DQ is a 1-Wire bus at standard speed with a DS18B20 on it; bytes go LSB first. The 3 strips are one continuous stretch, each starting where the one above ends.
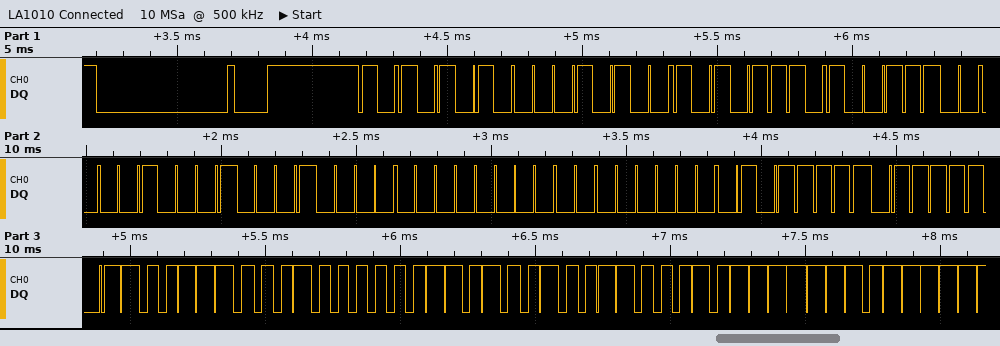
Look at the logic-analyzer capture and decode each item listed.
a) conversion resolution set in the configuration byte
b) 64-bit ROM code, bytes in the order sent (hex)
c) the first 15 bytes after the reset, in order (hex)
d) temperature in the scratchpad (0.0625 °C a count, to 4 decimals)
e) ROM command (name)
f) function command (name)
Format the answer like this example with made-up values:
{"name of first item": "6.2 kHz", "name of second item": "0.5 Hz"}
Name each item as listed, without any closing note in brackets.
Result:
{"conversion resolution set in the configuration byte": "12 bits", "64-bit ROM code, bytes in the order sent": "28 75 39 88 08 00 00 FA", "the first 15 bytes after the reset, in order": "55 28 75 39 88 08 00 00 FA BE 39 02 4B 46 7F", "temperature in the scratchpad": "35.5625 °C", "ROM command": "Match ROM", "function command": "Read Scratchpad"}
